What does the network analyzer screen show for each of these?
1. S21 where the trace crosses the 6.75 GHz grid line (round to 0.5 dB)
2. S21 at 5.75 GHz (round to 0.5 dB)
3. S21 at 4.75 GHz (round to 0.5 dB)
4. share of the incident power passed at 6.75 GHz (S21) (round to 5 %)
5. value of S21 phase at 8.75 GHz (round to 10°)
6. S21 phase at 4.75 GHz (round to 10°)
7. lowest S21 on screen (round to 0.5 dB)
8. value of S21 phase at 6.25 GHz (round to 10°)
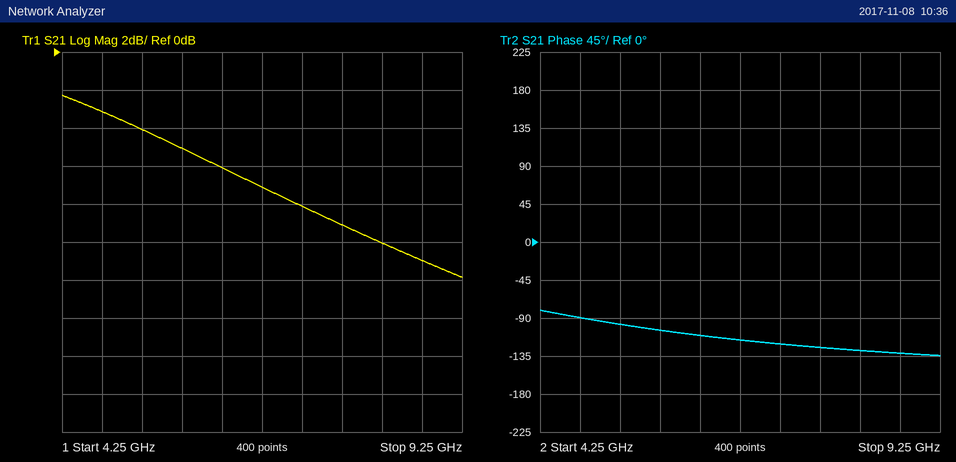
-7.0 dB
-5.0 dB
-3.0 dB
20 %
-130°
-90°
-12.0 dB
-110°
